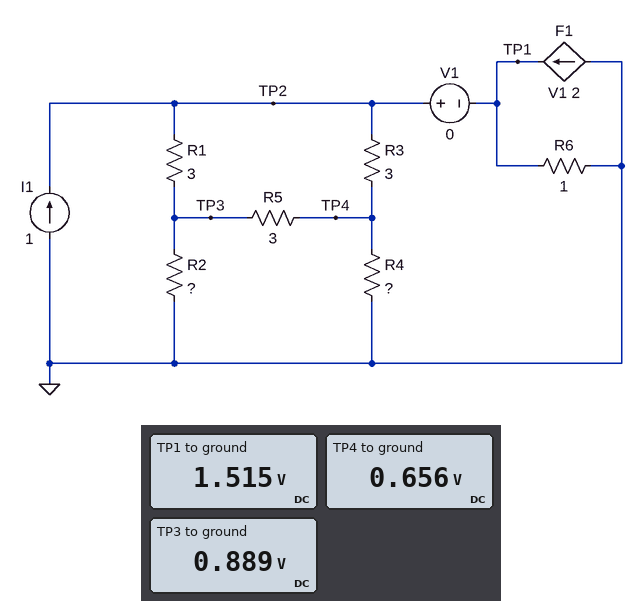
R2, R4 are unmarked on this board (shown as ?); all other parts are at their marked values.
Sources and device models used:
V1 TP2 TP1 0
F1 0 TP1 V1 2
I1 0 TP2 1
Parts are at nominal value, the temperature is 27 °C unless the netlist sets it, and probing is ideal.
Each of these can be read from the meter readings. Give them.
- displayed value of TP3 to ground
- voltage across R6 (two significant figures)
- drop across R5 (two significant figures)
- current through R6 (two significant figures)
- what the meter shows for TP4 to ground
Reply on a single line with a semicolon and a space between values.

0.889 V; 1.5 V; 230 mV; 1.5 A; 0.656 V
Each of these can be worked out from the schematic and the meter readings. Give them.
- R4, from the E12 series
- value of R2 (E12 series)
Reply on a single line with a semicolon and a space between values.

1.8 Ω; 6.8 Ω
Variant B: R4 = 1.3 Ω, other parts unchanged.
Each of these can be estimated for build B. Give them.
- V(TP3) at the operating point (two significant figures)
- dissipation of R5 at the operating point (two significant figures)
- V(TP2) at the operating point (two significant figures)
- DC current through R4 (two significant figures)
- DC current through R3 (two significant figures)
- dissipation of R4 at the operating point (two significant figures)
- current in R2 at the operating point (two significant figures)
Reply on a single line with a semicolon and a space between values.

800 mV; 27 mW; 1.4 V; 400 mA; 310 mA; 210 mW; 120 mA
